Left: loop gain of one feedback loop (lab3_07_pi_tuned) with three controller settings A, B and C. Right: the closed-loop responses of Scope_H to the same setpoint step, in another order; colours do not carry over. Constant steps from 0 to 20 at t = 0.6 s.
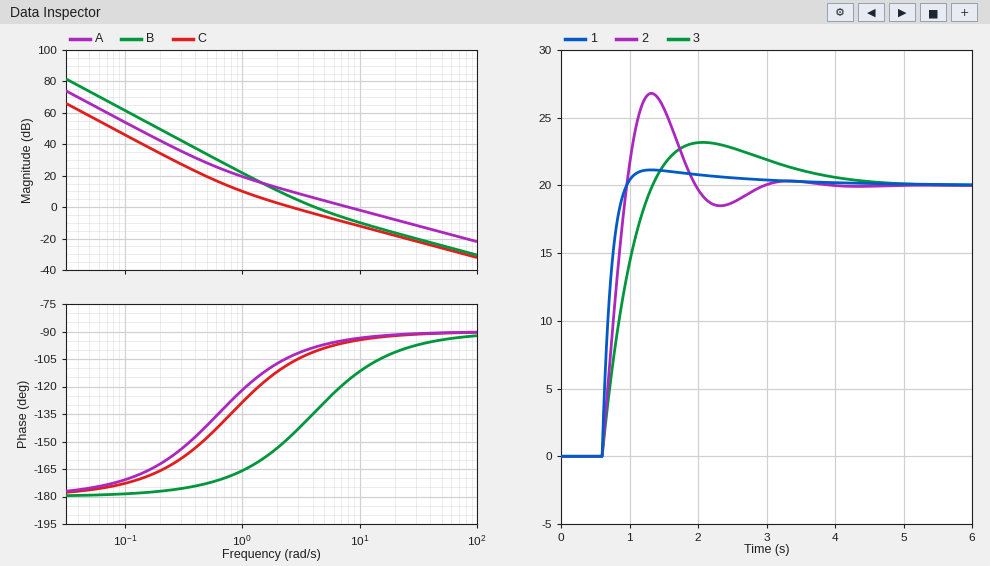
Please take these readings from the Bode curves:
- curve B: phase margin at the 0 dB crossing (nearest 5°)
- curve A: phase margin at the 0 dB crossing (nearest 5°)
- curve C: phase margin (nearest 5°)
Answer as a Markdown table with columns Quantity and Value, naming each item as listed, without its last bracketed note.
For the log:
| Quantity | Value |
|---|---|
| curve B: phase margin at the 0 dB crossing | 45° |
| curve A: phase margin at the 0 dB crossing | 85° |
| curve C: phase margin | 75° |
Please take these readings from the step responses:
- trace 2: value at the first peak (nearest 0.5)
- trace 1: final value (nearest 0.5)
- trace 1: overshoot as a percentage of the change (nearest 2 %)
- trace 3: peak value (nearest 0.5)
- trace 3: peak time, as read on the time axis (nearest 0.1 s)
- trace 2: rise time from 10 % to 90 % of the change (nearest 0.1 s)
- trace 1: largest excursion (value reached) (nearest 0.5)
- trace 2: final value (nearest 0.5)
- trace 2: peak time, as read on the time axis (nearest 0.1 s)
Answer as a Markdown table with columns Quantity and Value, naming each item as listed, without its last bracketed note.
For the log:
| Quantity | Value |
|---|---|
| trace 2: value at the first peak | 27.0 |
| trace 1: final value | 20.0 |
| trace 1: overshoot as a percentage of the change | 6 % |
| trace 3: peak value | 23.0 |
| trace 3: peak time, as read on the time axis | 2.1 s |
| trace 2: rise time from 10 % to 90 % of the change | 0.3 s |
| trace 1: largest excursion (value reached) | 21.0 |
| trace 2: final value | 20.0 |
| trace 2: peak time, as read on the time axis | 1.3 s |
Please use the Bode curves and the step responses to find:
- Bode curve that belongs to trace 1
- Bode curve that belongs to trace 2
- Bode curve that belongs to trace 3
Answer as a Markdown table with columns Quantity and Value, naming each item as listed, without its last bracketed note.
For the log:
| Quantity | Value |
|---|---|
| Bode curve that belongs to trace 1 | A |
| Bode curve that belongs to trace 2 | B |
| Bode curve that belongs to trace 3 | C |
